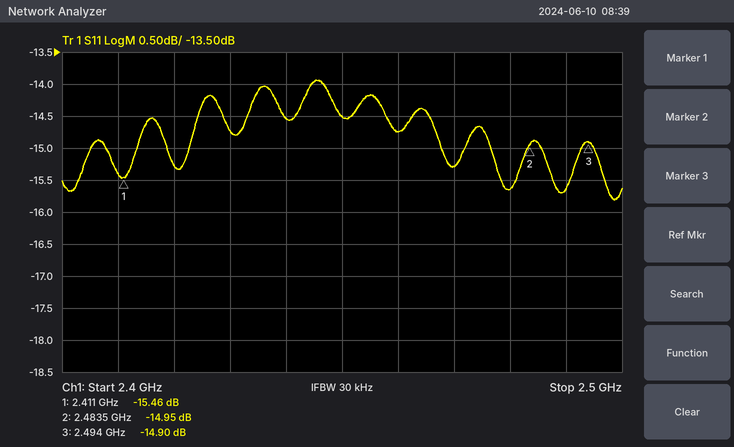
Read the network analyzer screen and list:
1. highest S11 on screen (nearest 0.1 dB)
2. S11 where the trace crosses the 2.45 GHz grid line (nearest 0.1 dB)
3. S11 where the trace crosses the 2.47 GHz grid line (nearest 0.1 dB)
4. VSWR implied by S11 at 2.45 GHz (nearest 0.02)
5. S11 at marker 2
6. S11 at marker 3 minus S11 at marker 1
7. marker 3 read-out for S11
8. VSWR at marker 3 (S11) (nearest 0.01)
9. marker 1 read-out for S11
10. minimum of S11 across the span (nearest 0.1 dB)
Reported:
-13.9 dB
-14.5 dB
-15.3 dB
1.46
-14.95 dB
0.56 dB
-14.90 dB
1.44
-15.46 dB
-15.8 dB
